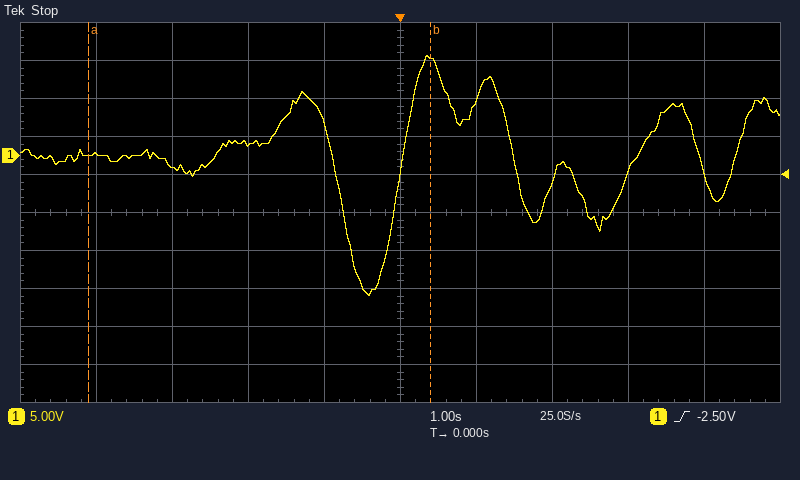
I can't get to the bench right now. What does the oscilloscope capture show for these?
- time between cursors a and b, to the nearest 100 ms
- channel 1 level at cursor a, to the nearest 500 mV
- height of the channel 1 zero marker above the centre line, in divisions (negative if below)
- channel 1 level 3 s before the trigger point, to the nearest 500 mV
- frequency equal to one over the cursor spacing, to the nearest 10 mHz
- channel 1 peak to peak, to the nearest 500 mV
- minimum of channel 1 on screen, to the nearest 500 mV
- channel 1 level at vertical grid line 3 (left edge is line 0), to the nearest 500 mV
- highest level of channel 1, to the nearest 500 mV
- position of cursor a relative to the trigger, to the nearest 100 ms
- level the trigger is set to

4.5 s
0.0 V
+1.5 div
-1.5 V
220 mHz
31.5 V
-18.5 V
1.5 V
13.0 V
-4.1 s
-2.50 V
